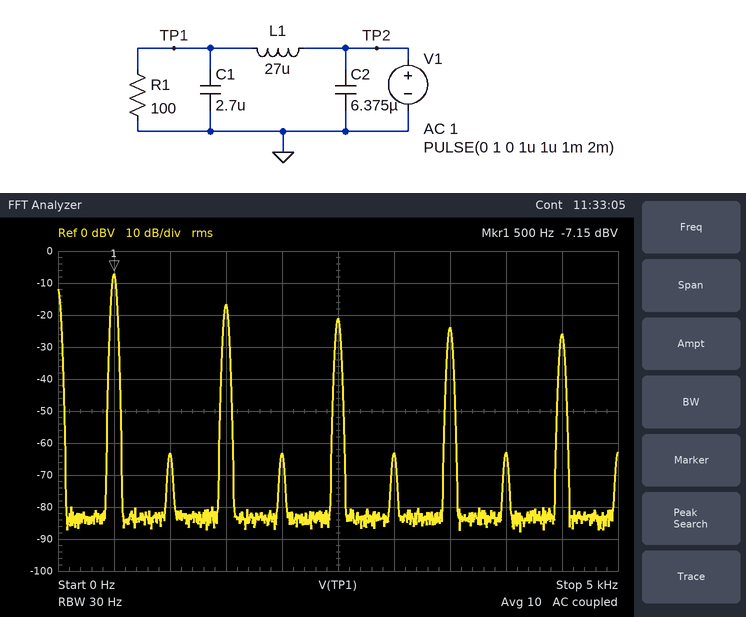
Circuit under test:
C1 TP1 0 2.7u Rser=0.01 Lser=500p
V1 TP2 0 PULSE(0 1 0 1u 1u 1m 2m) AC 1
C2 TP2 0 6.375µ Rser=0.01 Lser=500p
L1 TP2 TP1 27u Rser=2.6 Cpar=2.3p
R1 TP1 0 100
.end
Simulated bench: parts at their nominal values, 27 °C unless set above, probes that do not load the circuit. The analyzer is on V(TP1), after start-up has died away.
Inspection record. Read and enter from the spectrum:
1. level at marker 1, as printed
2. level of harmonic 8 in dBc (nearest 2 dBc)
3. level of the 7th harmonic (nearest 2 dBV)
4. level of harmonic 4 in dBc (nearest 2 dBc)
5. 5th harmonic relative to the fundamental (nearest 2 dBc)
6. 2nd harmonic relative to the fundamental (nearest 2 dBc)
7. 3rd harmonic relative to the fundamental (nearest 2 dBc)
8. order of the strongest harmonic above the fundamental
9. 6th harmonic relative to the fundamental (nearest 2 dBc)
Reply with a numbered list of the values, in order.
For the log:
1. -7.15 dBV
2. -56 dBc
3. -24 dBV
4. -56 dBc
5. -14 dBc
6. -56 dBc
7. -10 dBc
8. 3
9. -56 dBc
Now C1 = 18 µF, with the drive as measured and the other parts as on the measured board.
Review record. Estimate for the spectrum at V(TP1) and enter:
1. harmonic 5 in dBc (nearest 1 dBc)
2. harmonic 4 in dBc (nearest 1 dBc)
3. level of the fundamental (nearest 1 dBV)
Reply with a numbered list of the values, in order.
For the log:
1. -15 dBc
2. -57 dBc
3. -7 dBV
